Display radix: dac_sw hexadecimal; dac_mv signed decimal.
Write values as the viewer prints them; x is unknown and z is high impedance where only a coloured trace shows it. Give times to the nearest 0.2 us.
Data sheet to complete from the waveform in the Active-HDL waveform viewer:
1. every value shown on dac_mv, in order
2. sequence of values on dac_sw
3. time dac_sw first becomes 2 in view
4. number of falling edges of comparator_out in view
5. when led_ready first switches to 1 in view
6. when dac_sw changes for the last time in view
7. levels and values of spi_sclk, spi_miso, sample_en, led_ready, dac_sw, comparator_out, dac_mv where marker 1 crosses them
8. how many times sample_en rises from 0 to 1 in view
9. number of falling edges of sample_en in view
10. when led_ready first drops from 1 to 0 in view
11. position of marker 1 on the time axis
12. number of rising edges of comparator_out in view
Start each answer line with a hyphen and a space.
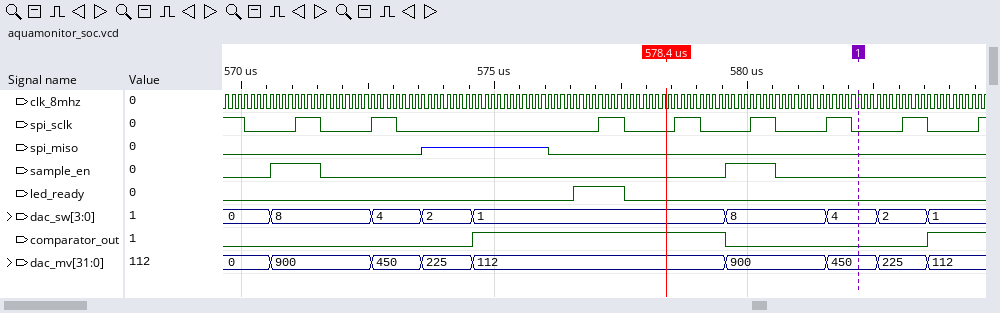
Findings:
- 0, 900, 450, 225, 112, 900, 450, 225, 112
- 0, 8, 4, 2, 1, 8, 4, 2, 1
- 573.6 us
- 1
- 576.6 us
- 583.6 us
- spi_sclk=0, spi_miso=0, sample_en=0, led_ready=0, dac_sw=4, comparator_out=0, dac_mv=450
- 2
- 2
- 577.6 us
- 582.2 us
- 2
